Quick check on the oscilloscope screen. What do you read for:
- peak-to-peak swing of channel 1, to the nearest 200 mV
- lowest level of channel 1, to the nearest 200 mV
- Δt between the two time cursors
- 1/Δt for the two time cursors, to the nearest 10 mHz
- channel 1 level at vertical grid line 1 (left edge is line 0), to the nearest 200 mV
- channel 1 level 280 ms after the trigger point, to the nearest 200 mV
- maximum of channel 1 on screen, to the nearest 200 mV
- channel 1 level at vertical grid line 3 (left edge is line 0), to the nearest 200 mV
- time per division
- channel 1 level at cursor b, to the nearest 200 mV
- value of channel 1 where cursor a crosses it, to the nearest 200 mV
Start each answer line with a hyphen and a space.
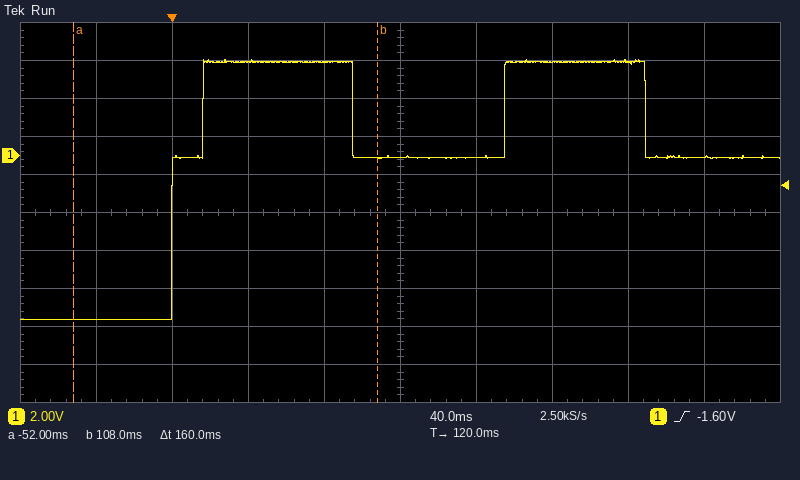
- 13.6 V
- -8.6 V
- 160 ms
- 6.25 Hz
- -8.6 V
- 0.0 V
- 5.0 V
- 5.0 V
- 40 ms
- -200 mV
- -8.6 V
